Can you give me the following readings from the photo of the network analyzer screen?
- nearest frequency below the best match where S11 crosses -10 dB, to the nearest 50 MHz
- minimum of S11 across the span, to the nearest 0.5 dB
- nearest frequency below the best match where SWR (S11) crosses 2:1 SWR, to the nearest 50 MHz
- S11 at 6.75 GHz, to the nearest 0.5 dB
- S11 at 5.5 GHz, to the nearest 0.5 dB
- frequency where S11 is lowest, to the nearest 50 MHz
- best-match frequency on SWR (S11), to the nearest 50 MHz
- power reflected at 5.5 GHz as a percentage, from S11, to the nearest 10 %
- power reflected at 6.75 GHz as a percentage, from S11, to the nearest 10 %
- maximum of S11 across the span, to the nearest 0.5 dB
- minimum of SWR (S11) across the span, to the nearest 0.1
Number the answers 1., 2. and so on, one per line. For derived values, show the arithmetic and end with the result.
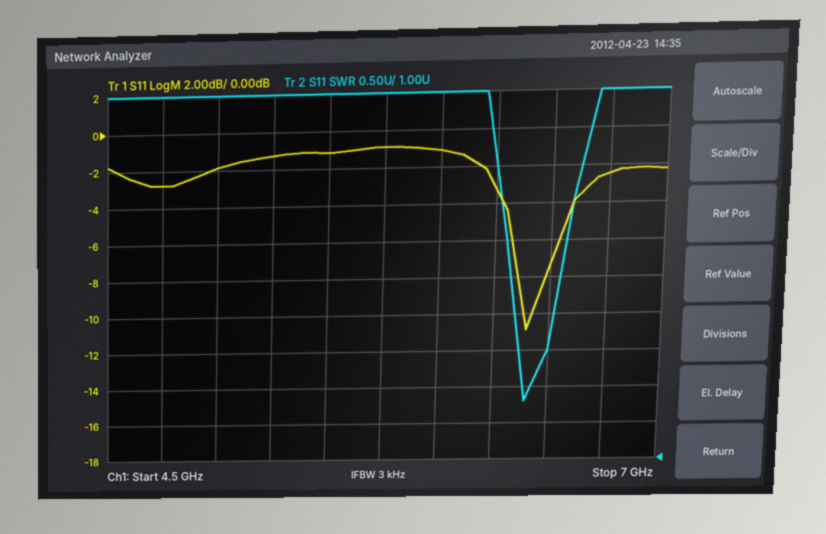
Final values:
1. 6.40 GHz
2. -11.0 dB
3. 6.40 GHz
4. -2.5 dB
5. -1.0 dB
6. 6.40 GHz
7. 6.40 GHz
8. 10^(-1/10) ≈ 79.4 %, so 80 % to the nearest 10 %
9. 10^(-2.5/10) ≈ 56.2 %, so 60 % to the nearest 10 %
10. -1.0 dB
11. 1.8
